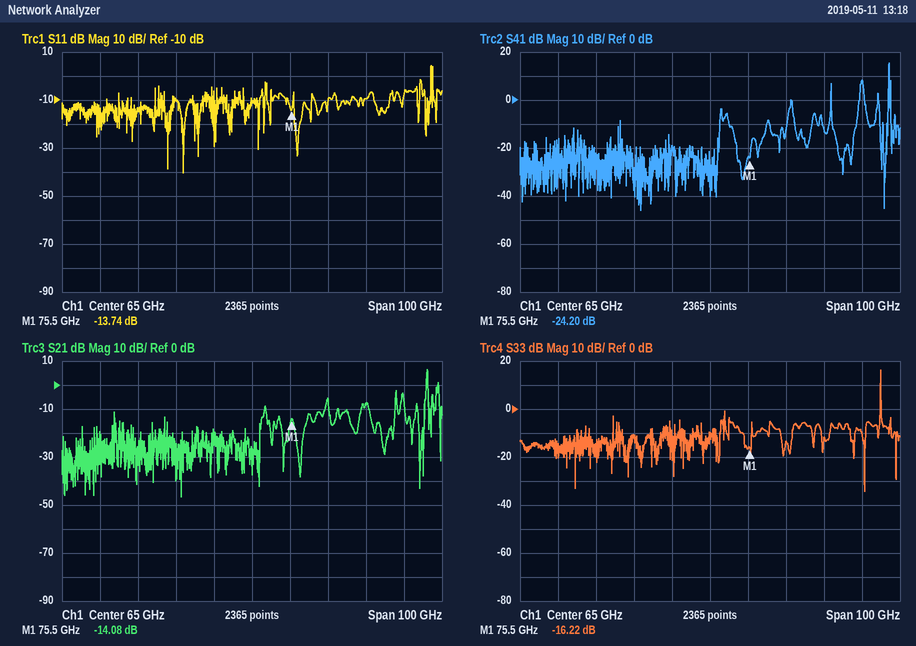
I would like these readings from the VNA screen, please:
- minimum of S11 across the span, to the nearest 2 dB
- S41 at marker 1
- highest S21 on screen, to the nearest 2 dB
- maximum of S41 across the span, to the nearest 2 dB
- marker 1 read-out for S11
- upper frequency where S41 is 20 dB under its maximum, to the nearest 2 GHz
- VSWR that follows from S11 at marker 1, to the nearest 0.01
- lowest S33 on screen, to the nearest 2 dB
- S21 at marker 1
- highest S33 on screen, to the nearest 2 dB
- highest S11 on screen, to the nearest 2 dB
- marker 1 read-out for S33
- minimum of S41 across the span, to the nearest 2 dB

-40 dB
-24.20 dB
6 dB
16 dB
-13.74 dB
112 GHz
1.52
-34 dB
-14.08 dB
16 dB
4 dB
-16.22 dB
-46 dB
